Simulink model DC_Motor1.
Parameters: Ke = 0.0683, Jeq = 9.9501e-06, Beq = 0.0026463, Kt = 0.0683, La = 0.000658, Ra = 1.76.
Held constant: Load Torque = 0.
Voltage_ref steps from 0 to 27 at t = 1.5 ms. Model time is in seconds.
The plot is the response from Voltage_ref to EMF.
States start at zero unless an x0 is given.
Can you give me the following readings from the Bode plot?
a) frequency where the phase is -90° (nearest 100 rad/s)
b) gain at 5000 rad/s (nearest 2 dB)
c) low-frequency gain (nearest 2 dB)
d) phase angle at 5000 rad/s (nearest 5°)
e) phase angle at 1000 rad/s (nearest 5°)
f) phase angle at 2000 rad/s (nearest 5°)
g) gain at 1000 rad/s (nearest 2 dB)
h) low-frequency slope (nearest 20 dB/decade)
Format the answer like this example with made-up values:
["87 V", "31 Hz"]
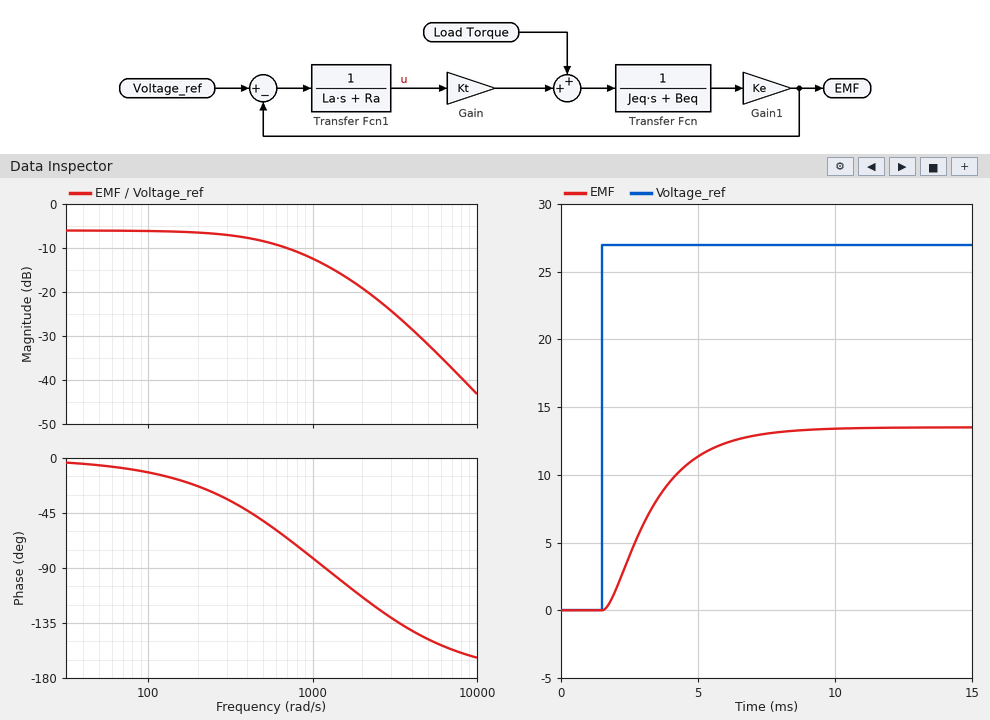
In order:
["1200 rad/s", "-32 dB", "-6 dB", "-150°", "-80°", "-115°", "-12 dB", "0 dB/decade"]
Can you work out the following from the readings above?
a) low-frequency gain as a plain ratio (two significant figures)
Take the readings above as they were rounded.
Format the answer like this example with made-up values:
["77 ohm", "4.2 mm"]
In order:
["0.50"]
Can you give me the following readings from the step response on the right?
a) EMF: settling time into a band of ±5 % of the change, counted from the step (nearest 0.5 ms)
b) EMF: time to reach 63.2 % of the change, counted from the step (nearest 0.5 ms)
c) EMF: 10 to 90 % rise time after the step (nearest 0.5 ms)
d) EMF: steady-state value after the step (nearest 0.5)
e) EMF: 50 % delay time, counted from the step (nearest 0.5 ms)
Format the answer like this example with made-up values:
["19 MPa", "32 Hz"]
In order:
["5.5 ms", "2.0 ms", "4.0 ms", "13.5", "1.5 ms"]
